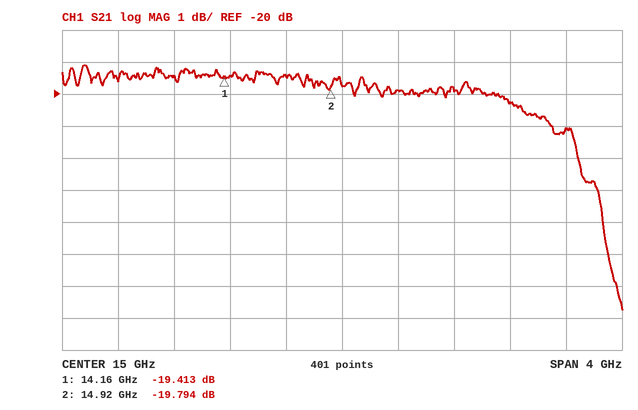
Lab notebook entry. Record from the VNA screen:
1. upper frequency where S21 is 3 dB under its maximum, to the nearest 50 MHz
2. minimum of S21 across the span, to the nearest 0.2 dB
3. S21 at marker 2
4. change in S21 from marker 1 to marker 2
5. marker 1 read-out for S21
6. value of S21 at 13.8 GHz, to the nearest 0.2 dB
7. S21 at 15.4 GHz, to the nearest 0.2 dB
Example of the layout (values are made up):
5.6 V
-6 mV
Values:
16.70 GHz
-26.8 dB
-19.794 dB
-0.381 dB
-19.413 dB
-19.4 dB
-19.8 dB
